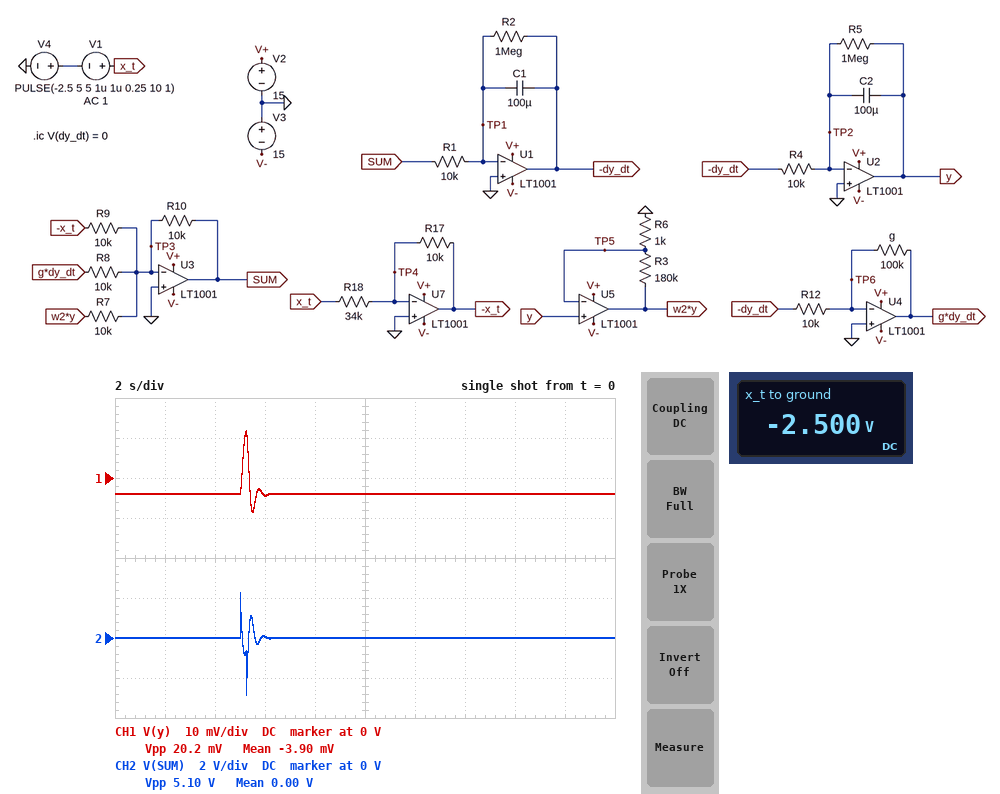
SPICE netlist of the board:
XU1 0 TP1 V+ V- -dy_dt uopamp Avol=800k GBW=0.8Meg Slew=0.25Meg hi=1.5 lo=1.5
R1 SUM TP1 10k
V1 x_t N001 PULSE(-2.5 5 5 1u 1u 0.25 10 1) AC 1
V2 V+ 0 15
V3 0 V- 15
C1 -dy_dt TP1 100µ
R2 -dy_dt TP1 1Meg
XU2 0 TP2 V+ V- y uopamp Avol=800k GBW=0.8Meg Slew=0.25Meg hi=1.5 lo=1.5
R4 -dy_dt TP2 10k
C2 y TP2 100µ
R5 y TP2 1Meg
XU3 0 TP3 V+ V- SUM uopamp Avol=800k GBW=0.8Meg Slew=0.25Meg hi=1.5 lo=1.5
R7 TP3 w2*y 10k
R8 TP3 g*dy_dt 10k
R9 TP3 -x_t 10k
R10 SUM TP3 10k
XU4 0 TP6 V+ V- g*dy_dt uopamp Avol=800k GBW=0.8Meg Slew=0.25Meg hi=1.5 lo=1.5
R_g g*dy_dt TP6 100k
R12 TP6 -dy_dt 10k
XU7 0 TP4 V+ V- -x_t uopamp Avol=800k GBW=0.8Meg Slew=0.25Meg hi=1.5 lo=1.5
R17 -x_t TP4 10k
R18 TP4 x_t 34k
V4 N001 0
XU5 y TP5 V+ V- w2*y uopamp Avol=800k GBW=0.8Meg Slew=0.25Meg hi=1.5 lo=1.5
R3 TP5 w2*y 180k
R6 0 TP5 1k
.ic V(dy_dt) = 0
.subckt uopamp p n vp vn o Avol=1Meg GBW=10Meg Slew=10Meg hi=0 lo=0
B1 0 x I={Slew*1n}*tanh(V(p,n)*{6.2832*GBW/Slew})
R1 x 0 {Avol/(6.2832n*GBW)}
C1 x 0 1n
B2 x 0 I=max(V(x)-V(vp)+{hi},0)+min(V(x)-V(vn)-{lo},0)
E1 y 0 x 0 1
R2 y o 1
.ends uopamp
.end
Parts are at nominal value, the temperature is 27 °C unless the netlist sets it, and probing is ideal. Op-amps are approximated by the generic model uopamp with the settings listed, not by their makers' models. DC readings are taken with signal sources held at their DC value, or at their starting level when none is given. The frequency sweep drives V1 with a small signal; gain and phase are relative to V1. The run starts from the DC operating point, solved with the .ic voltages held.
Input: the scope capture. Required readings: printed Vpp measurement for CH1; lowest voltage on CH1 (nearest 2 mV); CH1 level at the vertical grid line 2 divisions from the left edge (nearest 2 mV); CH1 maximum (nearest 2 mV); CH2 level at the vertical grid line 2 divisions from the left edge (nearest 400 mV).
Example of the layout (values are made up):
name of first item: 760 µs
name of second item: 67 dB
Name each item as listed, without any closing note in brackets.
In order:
printed Vpp measurement for CH1: 20.2 mV
lowest voltage on CH1: -8 mV
CH1 level at the vertical grid line 2 divisions from the left edge: -4 mV
CH1 maximum: 12 mV
CH2 level at the vertical grid line 2 divisions from the left edge: 0 V
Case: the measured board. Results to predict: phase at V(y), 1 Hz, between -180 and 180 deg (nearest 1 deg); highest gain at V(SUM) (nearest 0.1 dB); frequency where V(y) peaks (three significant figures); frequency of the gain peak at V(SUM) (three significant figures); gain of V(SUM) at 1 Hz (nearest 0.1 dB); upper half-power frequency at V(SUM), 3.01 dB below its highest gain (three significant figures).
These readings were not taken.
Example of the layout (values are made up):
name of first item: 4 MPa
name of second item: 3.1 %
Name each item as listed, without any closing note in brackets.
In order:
phase at V(y), 1 Hz, between -180 and 180 deg: -24 deg
highest gain at V(SUM): -7.4 dB
frequency where V(y) peaks: 1.82 Hz
frequency of the gain peak at V(SUM): 2.52 Hz
gain of V(SUM) at 1 Hz: -22.5 dB
upper half-power frequency at V(SUM), 3.01 dB below its highest gain: 11.9 Hz
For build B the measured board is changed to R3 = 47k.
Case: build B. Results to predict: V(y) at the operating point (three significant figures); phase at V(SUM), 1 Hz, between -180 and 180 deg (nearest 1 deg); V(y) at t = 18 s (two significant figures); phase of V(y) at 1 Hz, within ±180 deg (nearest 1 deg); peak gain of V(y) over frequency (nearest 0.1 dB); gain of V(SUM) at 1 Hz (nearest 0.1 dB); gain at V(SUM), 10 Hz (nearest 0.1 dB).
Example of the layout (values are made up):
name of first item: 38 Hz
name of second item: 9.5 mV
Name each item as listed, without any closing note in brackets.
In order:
V(y) at the operating point: -15.3 mV
phase at V(SUM), 1 Hz, between -180 and 180 deg: 98 deg
V(y) at t = 18 s: -15 mV
phase of V(y) at 1 Hz, within ±180 deg: -82 deg
peak gain of V(y) over frequency: -44.3 dB
gain of V(SUM) at 1 Hz: -14.8 dB
gain at V(SUM), 10 Hz: -10.6 dB
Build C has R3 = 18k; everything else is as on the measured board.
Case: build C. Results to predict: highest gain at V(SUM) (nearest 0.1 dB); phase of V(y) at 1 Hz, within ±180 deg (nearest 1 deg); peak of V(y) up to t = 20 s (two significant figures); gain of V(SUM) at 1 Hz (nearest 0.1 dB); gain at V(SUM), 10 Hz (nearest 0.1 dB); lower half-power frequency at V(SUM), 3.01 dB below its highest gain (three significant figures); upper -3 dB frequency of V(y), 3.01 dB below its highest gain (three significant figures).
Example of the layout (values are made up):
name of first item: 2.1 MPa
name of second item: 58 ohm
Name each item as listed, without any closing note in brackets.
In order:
highest gain at V(SUM): -10.6 dB
phase of V(y) at 1 Hz, within ±180 deg: -108 deg
peak of V(y) up to t = 20 s: 1.8 mV
gain of V(SUM) at 1 Hz: -15.1 dB
gain at V(SUM), 10 Hz: -10.7 dB
lower half-power frequency at V(SUM), 3.01 dB below its highest gain: 1.31 Hz
upper -3 dB frequency of V(y), 3.01 dB below its highest gain: 370 mHz
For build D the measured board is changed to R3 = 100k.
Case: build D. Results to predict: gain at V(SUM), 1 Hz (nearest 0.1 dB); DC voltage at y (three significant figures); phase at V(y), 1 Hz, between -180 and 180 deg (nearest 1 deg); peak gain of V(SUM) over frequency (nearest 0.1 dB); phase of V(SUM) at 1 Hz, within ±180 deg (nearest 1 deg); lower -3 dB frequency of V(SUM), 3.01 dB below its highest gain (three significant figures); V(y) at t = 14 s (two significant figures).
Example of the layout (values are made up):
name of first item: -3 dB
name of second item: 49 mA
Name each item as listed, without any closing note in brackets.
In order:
gain at V(SUM), 1 Hz: -17.6 dB
DC voltage at y: -7.27 mV
phase at V(y), 1 Hz, between -180 and 180 deg: -46 deg
peak gain of V(SUM) over frequency: -9.4 dB
phase of V(SUM) at 1 Hz, within ±180 deg: 134 deg
lower -3 dB frequency of V(SUM), 3.01 dB below its highest gain: 1.37 Hz
V(y) at t = 14 s: -7.3 mV
